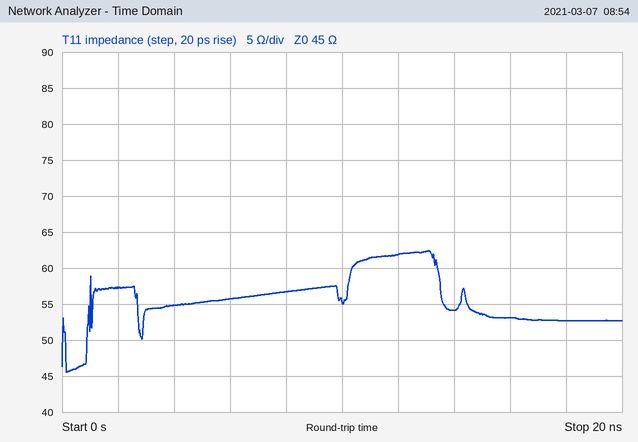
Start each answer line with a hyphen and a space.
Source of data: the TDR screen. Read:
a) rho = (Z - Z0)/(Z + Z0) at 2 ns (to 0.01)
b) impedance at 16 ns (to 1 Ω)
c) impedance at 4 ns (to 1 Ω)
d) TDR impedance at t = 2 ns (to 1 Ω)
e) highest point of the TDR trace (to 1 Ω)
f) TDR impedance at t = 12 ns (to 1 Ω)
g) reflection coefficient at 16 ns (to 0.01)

- +0.12
- 53 Ω
- 55 Ω
- 57 Ω
- 62 Ω
- 62 Ω
- +0.08
